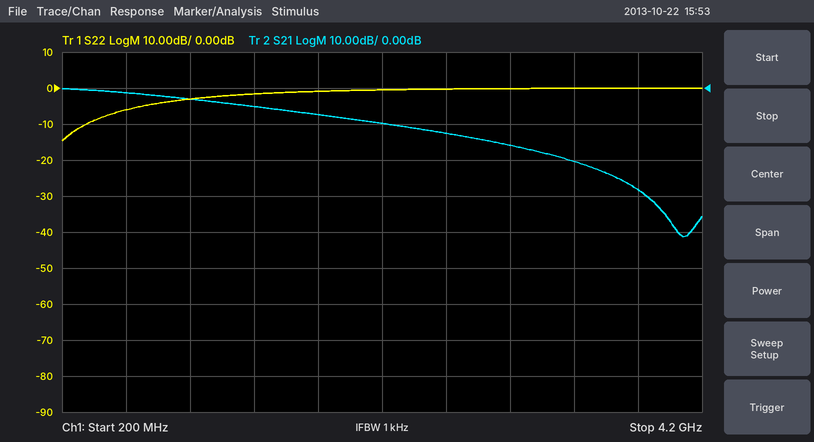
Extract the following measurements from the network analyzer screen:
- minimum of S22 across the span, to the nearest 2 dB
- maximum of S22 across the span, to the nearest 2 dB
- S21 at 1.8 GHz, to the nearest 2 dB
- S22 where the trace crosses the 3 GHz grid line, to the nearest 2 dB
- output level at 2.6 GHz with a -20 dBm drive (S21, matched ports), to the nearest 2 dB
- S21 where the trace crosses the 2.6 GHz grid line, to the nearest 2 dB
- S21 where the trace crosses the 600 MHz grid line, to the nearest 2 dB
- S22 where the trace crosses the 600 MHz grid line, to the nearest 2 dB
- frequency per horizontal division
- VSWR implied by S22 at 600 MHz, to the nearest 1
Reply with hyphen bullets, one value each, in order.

- -14 dB
- 0 dB
- -8 dB
- 0 dB
- -32 dBm
- -12 dB
- -2 dB
- -6 dB
- 400 MHz
- 3
